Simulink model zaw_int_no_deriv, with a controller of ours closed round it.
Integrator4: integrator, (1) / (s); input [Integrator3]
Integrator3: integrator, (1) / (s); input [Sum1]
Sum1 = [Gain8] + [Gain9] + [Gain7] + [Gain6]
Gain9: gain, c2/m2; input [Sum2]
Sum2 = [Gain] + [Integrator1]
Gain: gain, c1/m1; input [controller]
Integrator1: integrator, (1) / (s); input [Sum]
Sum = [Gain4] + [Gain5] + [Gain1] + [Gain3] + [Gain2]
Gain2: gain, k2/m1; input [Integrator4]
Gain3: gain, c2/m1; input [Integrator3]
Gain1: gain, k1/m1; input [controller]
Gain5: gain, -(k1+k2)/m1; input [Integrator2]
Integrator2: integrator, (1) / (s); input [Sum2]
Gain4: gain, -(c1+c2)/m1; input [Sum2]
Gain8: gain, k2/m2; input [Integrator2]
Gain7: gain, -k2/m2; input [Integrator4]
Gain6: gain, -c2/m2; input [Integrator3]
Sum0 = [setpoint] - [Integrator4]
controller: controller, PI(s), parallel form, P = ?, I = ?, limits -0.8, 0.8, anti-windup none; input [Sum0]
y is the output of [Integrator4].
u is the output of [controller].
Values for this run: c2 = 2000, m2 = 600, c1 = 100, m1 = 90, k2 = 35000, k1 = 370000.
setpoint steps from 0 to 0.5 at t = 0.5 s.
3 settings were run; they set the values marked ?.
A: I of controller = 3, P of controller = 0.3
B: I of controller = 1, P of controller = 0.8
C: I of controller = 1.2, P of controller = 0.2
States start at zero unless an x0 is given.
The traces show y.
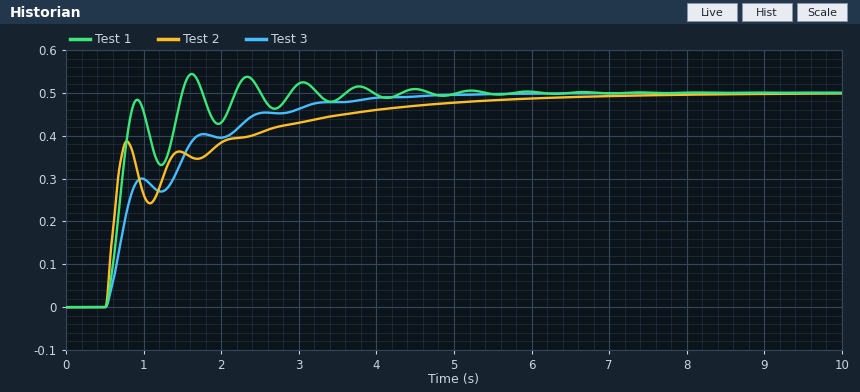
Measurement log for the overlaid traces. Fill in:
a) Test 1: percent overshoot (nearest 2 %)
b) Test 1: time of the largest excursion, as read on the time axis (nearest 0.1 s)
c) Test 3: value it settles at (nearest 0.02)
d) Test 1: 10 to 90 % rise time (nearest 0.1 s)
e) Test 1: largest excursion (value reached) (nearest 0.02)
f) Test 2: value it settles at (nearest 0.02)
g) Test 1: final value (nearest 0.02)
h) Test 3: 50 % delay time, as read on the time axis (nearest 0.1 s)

8 %
1.6 s
0.50
0.3 s
0.54
0.50
0.50
0.8 s
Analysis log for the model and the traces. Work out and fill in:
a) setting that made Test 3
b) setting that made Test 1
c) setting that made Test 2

C
A
B
